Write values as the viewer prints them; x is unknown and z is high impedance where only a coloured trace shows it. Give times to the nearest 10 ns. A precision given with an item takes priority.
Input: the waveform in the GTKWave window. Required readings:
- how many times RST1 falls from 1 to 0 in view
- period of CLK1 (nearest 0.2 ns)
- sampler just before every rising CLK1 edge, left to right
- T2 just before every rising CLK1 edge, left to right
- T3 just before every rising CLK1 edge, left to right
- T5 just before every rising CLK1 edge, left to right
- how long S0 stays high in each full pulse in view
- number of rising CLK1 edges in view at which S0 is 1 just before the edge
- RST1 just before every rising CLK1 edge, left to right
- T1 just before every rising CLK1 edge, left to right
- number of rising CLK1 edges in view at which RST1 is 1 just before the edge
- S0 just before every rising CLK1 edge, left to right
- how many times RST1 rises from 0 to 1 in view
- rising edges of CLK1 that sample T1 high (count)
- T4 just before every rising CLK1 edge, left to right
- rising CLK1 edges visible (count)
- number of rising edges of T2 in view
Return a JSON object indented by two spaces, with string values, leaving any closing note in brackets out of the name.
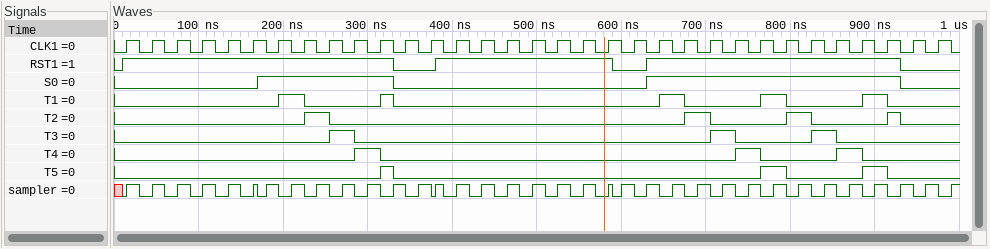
{
  "how many times RST1 falls from 1 to 0 in view": "3",
  "period of CLK1": "30 ns",
  "sampler just before every rising CLK1 edge, left to right": "0 0 0 0 0 0 1 1 1 1 1 1 1 0 0 0 0 0 0 0 1 1 1 1 1 1 1 1 1 1 1 1 1",
  "T2 just before every rising CLK1 edge, left to right": "0 0 0 0 0 0 0 0 1 0 0 0 0 0 0 0 0 0 0 0 0 0 0 1 0 0 0 1 0 0 0 0 0",
  "T3 just before every rising CLK1 edge, left to right": "0 0 0 0 0 0 0 0 0 1 0 0 0 0 0 0 0 0 0 0 0 0 0 0 1 0 0 0 1 0 0 0 0",
  "T5 just before every rising CLK1 edge, left to right": "0 0 0 0 0 0 0 0 0 0 0 0 0 0 0 0 0 0 0 0 0 0 0 0 0 0 1 0 0 0 1 0 0",
  "how long S0 stays high in each full pulse in view": "160 ns, 300 ns",
  "number of rising CLK1 edges in view at which S0 is 1 just before the edge": "15",
  "RST1 just before every rising CLK1 edge, left to right": "1 1 1 1 1 1 1 1 1 1 1 0 0 1 1 1 1 1 1 1 0 1 1 1 1 1 1 1 1 1 1 0 0",
  "T1 just before every rising CLK1 edge, left to right": "0 0 0 0 0 0 0 1 0 0 0 0 0 0 0 0 0 0 0 0 0 0 1 0 0 0 1 0 0 0 1 0 0",
  "number of rising CLK1 edges in view at which RST1 is 1 just before the edge": "28",
  "S0 just before every rising CLK1 edge, left to right": "0 0 0 0 0 0 1 1 1 1 1 0 0 0 0 0 0 0 0 0 0 1 1 1 1 1 1 1 1 1 1 0 0",
  "how many times RST1 rises from 0 to 1 in view": "3",
  "rising edges of CLK1 that sample T1 high": "4",
  "T4 just before every rising CLK1 edge, left to right": "0 0 0 0 0 0 0 0 0 0 1 0 0 0 0 0 0 0 0 0 0 0 0 0 0 1 0 0 0 1 0 0 0",
  "rising CLK1 edges visible": "33",
  "number of rising edges of T2 in view": "4"
}
